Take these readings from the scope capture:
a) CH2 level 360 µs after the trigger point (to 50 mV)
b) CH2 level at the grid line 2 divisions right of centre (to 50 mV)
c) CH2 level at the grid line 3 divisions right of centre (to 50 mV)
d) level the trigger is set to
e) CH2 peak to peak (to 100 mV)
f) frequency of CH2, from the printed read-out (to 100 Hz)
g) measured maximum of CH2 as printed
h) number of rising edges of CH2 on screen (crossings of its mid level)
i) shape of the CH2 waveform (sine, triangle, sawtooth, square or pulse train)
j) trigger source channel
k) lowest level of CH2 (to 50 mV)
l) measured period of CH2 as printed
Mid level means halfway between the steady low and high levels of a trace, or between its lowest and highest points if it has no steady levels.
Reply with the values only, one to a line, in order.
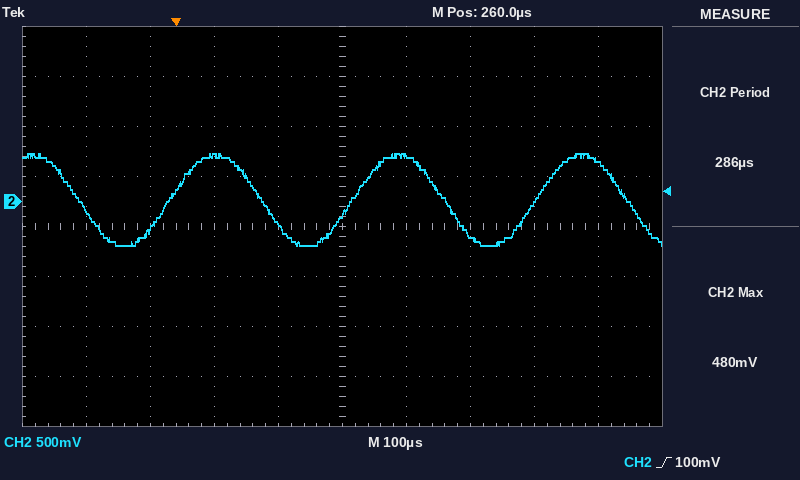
450 mV
-350 mV
0 mV
100 mV
900 mV
3.5 kHz
480 mV
3
sine
CH2
-450 mV
286 µs
